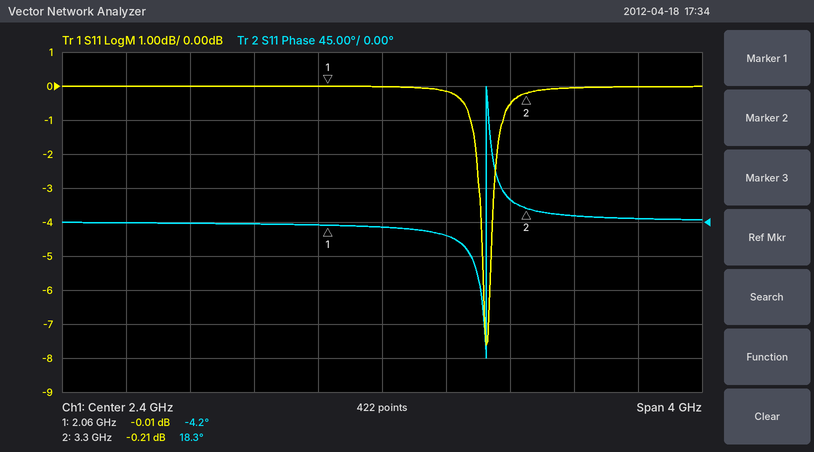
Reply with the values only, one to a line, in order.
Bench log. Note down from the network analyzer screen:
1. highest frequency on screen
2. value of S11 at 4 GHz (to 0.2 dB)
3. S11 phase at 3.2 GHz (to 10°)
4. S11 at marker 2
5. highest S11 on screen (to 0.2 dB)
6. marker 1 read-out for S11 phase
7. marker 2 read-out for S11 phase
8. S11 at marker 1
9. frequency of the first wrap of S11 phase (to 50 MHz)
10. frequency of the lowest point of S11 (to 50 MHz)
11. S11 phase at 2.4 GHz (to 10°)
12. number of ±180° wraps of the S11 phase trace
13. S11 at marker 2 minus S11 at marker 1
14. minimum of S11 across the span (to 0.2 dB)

4.4 GHz
0.0 dB
30°
-0.21 dB
0.0 dB
-4.2°
18.3°
-0.01 dB
3.05 GHz
3.05 GHz
-10°
1
-0.20 dB
-7.6 dB
